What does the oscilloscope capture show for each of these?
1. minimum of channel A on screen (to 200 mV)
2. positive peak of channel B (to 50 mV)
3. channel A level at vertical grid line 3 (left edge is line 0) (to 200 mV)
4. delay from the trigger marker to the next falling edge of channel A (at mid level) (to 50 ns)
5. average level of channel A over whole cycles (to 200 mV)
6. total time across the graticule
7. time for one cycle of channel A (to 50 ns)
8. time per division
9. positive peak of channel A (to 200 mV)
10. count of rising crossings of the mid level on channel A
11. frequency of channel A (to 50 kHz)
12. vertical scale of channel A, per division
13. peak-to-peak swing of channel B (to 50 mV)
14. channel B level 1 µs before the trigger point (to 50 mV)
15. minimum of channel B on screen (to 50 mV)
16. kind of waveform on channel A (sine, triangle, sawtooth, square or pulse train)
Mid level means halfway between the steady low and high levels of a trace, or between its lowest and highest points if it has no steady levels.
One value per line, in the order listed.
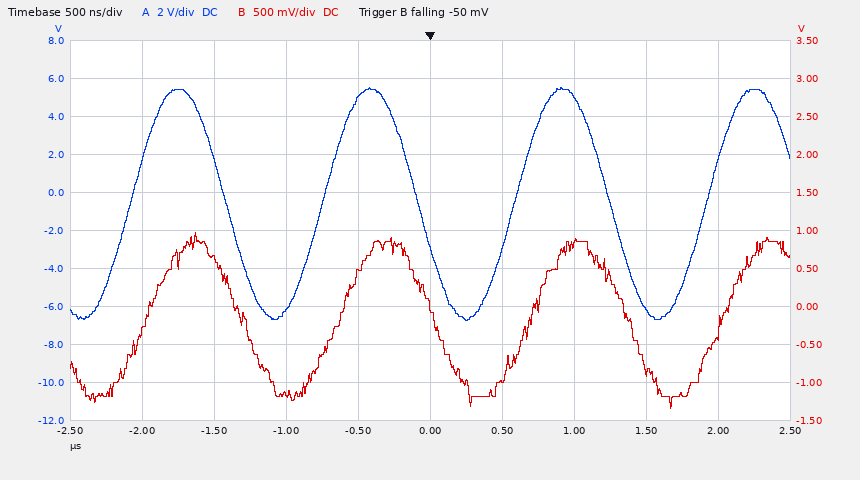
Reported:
-6.8 V
950 mV
-6.2 V
1.25 µs
-600 mV
5 µs
1.35 µs
500 ns
5.6 V
4
750 kHz
2 V
2.30 V
-1.15 V
-1.35 V
sine
